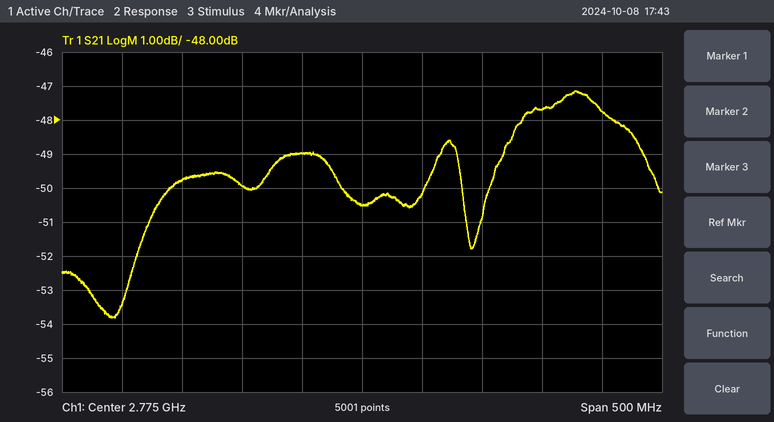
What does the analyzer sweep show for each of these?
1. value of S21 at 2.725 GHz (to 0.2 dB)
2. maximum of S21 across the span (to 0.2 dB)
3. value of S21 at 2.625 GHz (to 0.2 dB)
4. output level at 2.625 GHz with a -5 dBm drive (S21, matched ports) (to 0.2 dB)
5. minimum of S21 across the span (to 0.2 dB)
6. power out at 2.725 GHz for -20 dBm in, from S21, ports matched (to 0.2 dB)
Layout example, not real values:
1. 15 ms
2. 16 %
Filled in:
1. -49.0 dB
2. -47.2 dB
3. -49.8 dB
4. -54.8 dBm
5. -53.8 dB
6. -69.0 dBm
